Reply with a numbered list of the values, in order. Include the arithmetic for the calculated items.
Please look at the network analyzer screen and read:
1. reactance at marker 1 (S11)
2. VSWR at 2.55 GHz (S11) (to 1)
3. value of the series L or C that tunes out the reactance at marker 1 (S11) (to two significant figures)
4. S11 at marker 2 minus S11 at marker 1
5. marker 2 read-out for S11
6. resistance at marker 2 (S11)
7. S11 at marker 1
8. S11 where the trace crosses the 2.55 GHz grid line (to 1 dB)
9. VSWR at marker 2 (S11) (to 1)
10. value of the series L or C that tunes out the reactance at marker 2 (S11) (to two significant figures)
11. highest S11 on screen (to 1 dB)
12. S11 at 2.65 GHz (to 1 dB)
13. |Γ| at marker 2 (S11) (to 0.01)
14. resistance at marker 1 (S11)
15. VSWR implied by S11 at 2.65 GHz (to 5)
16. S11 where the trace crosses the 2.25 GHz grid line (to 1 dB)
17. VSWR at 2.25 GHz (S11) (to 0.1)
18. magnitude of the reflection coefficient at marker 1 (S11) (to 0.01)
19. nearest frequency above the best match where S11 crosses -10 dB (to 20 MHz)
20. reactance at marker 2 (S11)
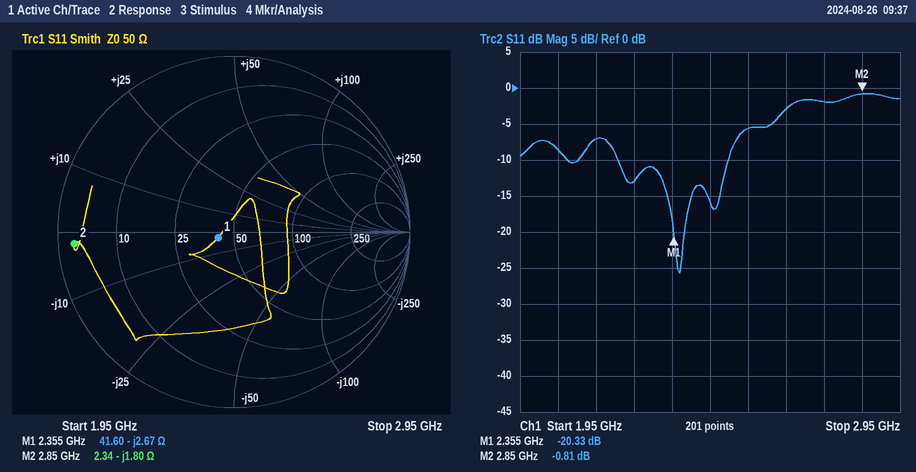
1. -2.67 Ω
2. |Γ| = 10^(-6/20) = 0.5012; VSWR = (1 + 0.5012)/(1 − 0.5012) ≈ 3
3. L = 2.67 Ω/(2π × 2.355 GHz) ≈ 180 pH
4. -0.81 − (-20.33) = 19.52 dB
5. -0.81 dB
6. 2.34 Ω
7. -20.33 dB
8. -6 dB
9. (1 + 0.9110)/(1 − 0.9110) ≈ 21
10. L = 1.8 Ω/(2π × 2.85 GHz) ≈ 101 pH, so 100 pH to two significant figures
11. -1 dB
12. -3 dB
13. 0.91
14. 41.60 Ω
15. |Γ| = 10^(-3/20) = 0.7079; VSWR = (1 + 0.7079)/(1 − 0.7079) ≈ 5.85, so 5 to the nearest 5
16. -13 dB
17. |Γ| = 10^(-13/20) = 0.2239; VSWR = (1 + 0.2239)/(1 − 0.2239) ≈ 1.6
18. 0.10
19. 2.50 GHz
20. -1.80 Ω
